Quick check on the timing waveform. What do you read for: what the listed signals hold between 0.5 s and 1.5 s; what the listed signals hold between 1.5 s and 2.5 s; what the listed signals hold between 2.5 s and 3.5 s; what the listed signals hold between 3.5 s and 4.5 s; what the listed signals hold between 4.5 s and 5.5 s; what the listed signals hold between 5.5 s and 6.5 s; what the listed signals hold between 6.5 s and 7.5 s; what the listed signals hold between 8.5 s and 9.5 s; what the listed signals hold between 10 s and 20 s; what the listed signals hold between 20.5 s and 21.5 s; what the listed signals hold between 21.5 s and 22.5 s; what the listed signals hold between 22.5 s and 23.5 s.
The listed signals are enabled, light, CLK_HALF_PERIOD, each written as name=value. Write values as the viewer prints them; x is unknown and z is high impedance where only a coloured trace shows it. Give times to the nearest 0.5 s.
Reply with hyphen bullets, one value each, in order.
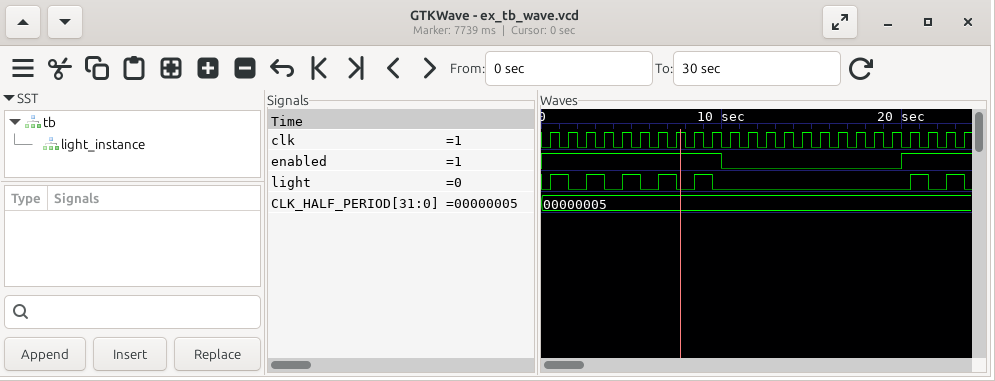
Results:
- enabled=1, light=1, CLK_HALF_PERIOD=00000005
- enabled=1, light=0, CLK_HALF_PERIOD=00000005
- enabled=1, light=1, CLK_HALF_PERIOD=00000005
- enabled=1, light=0, CLK_HALF_PERIOD=00000005
- enabled=1, light=1, CLK_HALF_PERIOD=00000005
- enabled=1, light=0, CLK_HALF_PERIOD=00000005
- enabled=1, light=1, CLK_HALF_PERIOD=00000005
- enabled=1, light=1, CLK_HALF_PERIOD=00000005
- enabled=0, light=0, CLK_HALF_PERIOD=00000005
- enabled=1, light=1, CLK_HALF_PERIOD=00000005
- enabled=1, light=0, CLK_HALF_PERIOD=00000005
- enabled=1, light=1, CLK_HALF_PERIOD=00000005
